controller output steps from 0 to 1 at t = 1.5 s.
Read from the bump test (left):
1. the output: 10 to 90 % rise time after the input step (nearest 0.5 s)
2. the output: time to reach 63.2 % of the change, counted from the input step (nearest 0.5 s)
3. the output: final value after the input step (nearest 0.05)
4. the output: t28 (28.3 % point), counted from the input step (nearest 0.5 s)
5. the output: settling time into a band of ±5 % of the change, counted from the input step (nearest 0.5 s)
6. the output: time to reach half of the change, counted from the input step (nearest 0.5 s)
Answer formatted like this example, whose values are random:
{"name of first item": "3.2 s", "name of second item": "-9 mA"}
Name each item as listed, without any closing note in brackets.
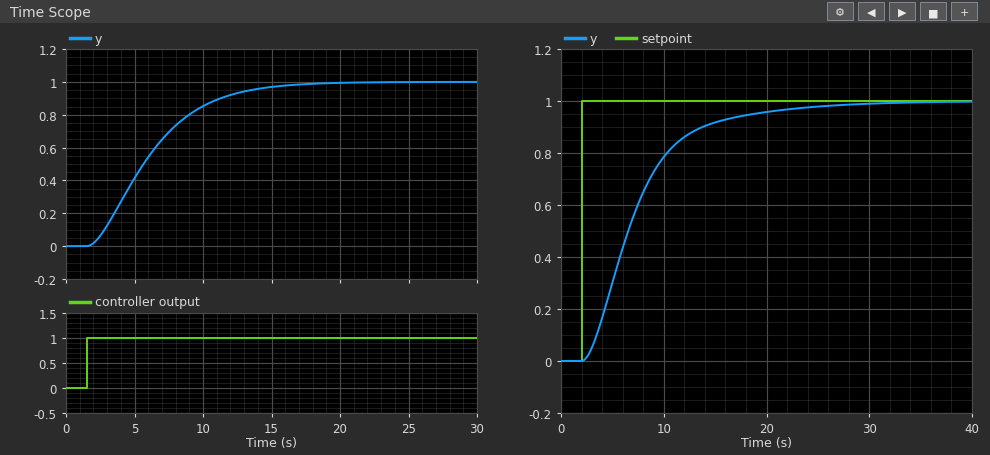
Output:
{"the output: 10 to 90 % rise time after the input step": "8.5 s", "the output: time to reach 63.2 % of the change, counted from the input step": "5.5 s", "the output: final value after the input step": "1.00", "the output: t28 (28.3 % point), counted from the input step": "2.5 s", "the output: settling time into a band of ±5 % of the change, counted from the input step": "12.0 s", "the output: time to reach half of the change, counted from the input step": "4.0 s"}
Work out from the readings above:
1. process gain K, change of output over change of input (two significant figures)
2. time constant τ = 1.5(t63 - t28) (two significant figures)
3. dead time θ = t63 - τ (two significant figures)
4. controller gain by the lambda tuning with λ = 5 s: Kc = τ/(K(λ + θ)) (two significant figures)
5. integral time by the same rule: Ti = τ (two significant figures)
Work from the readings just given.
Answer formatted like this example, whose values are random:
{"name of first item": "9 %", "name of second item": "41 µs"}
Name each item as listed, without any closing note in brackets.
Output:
{"process gain K, change of output over change of input": "1.0", "time constant τ = 1.5(t63 - t28)": "4.5 s", "dead time θ = t63 - τ": "1.0 s", "controller gain by the lambda tuning with λ = 5 s: Kc = τ/(K(λ + θ))": "0.75", "integral time by the same rule: Ti = τ": "4.5 s"}
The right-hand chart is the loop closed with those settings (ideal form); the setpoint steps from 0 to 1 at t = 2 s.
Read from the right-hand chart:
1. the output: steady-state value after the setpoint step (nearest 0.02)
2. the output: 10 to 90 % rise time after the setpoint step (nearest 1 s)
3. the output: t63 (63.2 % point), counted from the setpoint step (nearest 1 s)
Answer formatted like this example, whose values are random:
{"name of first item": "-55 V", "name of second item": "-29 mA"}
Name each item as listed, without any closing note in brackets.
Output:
{"the output: steady-state value after the setpoint step": "1.00", "the output: 10 to 90 % rise time after the setpoint step": "10 s", "the output: t63 (63.2 % point), counted from the setpoint step": "6 s"}
